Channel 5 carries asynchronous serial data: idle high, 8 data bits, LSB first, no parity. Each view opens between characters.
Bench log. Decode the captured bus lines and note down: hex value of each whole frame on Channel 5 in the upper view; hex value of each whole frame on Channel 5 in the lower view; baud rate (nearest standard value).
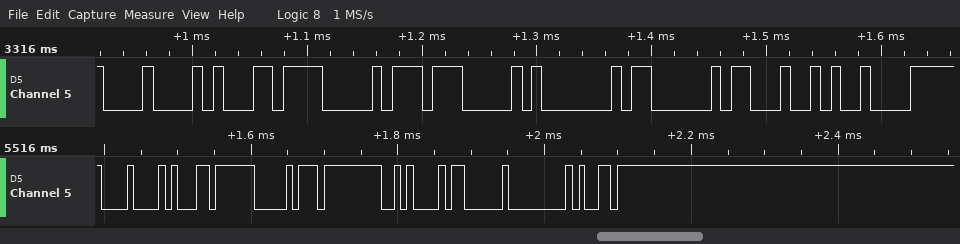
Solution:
08, B1, D0, 07, 01, 03, 23, 09
08, B1, D0, FF, 0A, 03, 00, D9
115200 baud
